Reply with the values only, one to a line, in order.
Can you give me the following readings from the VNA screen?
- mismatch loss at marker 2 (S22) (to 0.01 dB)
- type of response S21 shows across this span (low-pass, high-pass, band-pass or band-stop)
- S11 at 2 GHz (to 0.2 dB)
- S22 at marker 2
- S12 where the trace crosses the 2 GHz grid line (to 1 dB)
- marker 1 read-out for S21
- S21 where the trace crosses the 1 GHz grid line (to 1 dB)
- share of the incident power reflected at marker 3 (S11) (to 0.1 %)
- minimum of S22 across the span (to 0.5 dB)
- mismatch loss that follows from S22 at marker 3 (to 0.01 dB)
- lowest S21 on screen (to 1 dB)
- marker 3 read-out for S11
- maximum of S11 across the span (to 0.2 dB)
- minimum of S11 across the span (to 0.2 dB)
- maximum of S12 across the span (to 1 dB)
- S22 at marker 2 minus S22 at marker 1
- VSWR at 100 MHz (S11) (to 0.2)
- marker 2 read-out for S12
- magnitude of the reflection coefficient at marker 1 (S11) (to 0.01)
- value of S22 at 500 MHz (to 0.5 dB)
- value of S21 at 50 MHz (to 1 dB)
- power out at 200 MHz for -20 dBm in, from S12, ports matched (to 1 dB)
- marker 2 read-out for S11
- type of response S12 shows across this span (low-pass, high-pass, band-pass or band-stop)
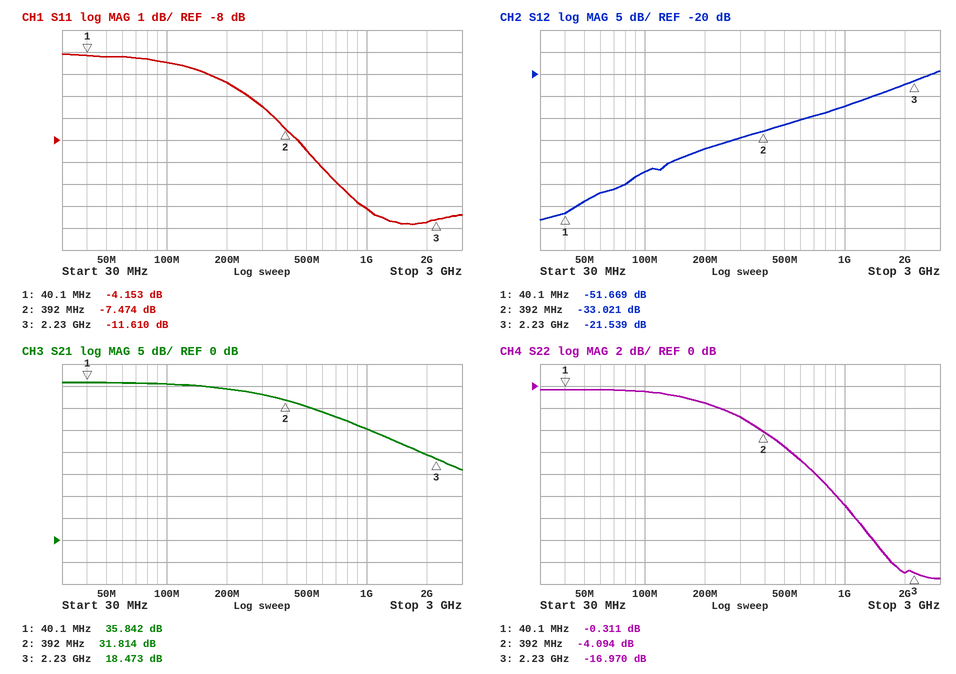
2.14 dB
low-pass
-11.8 dB
-4.094 dB
-22 dB
35.842 dB
25 dB
6.9 %
-17.5 dB
0.09 dB
16 dB
-11.610 dB
-4.0 dB
-11.8 dB
-19 dB
-3.783 dB
4.0
-33.021 dB
0.62
-5.5 dB
36 dB
-57 dBm
-7.474 dB
high-pass
